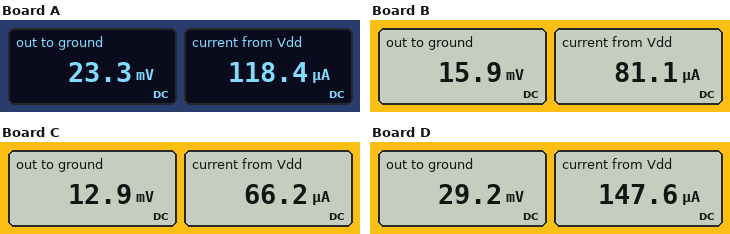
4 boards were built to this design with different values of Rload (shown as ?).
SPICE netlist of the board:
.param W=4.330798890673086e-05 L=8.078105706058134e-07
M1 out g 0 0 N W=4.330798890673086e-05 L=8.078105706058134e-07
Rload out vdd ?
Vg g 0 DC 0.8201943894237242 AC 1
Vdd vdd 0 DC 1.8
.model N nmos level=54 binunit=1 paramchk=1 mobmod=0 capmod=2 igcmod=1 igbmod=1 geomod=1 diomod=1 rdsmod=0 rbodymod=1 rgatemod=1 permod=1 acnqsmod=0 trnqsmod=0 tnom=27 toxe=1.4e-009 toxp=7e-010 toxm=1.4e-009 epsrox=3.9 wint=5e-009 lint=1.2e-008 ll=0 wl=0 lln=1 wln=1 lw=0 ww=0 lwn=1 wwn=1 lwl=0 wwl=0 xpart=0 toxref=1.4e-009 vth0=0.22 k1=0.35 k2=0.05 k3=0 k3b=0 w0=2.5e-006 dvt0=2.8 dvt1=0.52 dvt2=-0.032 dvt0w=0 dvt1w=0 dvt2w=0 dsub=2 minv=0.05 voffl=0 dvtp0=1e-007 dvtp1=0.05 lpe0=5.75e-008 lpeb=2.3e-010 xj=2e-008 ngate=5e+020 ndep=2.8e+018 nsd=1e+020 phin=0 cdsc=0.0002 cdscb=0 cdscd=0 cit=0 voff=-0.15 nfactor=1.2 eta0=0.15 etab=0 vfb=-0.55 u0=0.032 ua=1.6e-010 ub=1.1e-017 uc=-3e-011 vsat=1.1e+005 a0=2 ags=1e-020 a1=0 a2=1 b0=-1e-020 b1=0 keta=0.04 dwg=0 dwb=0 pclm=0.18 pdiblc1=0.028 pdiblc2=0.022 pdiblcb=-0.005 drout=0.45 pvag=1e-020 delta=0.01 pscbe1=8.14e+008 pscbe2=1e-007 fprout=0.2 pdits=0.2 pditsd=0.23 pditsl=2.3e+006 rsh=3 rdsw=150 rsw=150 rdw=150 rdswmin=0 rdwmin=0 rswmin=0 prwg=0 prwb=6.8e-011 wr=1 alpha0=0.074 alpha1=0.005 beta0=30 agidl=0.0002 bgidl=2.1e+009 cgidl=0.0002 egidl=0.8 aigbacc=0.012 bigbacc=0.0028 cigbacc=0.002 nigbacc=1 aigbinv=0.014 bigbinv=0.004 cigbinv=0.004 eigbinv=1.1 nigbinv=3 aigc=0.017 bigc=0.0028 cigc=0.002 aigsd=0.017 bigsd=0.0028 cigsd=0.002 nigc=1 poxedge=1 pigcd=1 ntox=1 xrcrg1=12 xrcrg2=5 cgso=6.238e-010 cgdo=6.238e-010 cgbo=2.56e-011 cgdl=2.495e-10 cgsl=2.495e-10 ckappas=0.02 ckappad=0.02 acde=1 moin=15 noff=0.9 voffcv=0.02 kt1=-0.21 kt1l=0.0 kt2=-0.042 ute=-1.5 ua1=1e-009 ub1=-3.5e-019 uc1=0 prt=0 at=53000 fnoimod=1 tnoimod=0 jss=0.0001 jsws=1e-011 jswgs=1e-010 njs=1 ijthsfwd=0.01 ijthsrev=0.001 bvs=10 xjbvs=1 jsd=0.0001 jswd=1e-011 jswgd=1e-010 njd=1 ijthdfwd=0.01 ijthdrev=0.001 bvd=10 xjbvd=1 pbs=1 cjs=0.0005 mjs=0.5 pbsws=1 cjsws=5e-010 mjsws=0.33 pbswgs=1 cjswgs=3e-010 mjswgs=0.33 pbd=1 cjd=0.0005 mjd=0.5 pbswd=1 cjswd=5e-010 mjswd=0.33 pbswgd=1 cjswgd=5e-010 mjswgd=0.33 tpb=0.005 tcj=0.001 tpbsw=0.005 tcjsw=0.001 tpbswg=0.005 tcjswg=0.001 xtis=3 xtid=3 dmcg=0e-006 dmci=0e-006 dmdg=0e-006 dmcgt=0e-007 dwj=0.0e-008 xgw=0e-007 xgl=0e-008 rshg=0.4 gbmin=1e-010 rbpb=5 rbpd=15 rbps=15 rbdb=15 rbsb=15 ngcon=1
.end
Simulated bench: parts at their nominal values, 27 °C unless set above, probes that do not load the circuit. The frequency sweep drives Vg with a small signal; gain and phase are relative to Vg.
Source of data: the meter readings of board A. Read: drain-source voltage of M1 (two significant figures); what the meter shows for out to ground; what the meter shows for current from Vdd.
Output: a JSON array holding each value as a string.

["23 mV", "23.3 mV", "118.4 µA"]
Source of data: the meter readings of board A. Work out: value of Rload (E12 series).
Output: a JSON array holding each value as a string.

["15 kΩ"]
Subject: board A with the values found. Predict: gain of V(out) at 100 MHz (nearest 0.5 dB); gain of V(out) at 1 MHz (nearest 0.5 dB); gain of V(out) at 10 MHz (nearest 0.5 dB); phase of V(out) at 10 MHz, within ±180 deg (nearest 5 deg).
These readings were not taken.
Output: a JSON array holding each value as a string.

["-21.0 dB", "-42.0 dB", "-38.5 dB", "130 deg"]
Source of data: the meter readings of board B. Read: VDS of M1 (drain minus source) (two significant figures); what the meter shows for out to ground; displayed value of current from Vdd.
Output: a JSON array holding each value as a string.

["16 mV", "15.9 mV", "81.1 µA"]
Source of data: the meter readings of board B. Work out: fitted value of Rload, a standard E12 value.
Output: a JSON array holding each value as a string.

["22 kΩ"]
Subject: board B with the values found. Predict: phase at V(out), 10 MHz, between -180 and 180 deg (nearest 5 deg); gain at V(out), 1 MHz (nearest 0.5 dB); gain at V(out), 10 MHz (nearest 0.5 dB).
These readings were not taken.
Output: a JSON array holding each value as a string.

["120 deg", "-46.0 dB", "-40.0 dB"]
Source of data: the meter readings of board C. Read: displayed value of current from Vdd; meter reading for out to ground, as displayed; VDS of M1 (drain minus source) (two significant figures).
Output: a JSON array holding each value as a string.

["66.2 µA", "12.9 mV", "13 mV"]
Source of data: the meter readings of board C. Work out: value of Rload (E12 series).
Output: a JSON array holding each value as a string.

["27 kΩ"]
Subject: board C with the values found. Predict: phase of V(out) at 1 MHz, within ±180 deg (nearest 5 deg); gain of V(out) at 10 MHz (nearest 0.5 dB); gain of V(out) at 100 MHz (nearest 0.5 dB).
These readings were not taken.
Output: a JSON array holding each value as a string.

["165 deg", "-40.5 dB", "-21.5 dB"]
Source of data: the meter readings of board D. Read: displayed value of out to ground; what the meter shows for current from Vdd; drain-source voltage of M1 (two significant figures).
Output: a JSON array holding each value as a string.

["29.2 mV", "147.6 µA", "29 mV"]
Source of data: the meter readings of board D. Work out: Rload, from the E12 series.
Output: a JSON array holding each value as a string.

["12 kΩ"]
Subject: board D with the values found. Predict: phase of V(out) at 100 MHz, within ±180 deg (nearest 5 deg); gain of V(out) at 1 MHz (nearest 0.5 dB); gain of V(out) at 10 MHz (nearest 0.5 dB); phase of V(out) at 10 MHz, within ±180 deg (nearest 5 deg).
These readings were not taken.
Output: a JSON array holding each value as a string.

["90 deg", "-39.5 dB", "-37.5 dB", "140 deg"]
